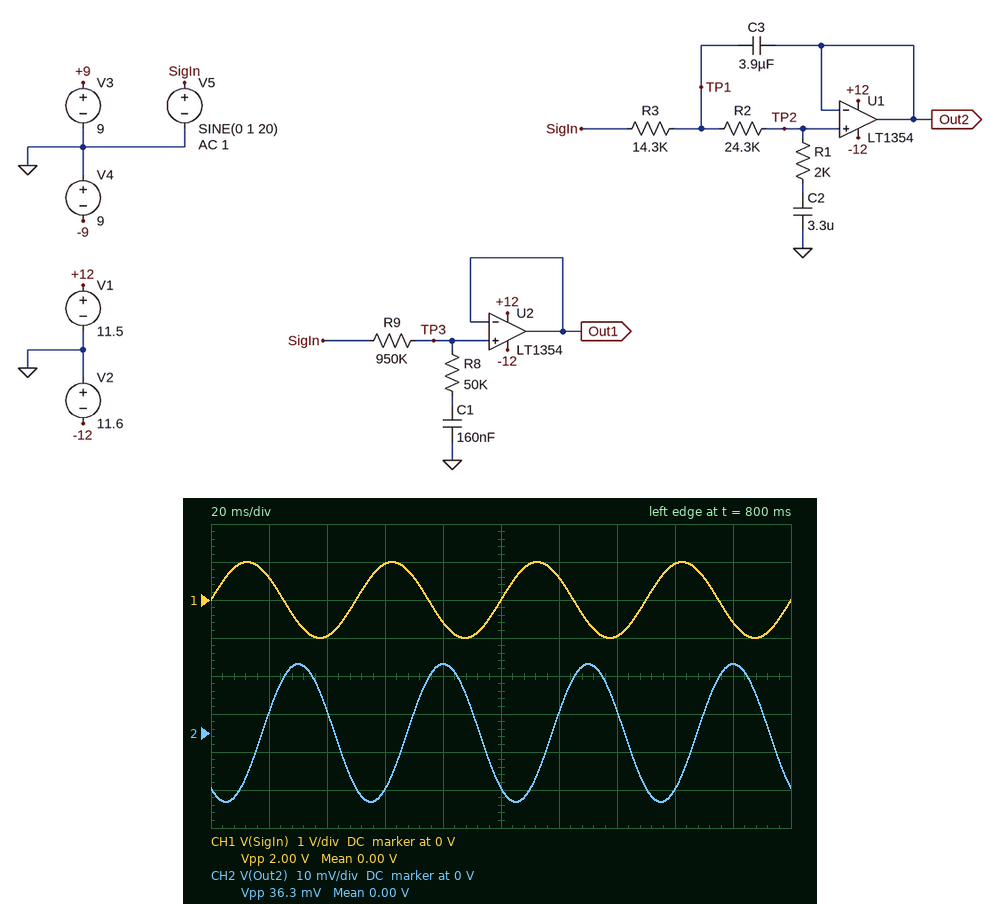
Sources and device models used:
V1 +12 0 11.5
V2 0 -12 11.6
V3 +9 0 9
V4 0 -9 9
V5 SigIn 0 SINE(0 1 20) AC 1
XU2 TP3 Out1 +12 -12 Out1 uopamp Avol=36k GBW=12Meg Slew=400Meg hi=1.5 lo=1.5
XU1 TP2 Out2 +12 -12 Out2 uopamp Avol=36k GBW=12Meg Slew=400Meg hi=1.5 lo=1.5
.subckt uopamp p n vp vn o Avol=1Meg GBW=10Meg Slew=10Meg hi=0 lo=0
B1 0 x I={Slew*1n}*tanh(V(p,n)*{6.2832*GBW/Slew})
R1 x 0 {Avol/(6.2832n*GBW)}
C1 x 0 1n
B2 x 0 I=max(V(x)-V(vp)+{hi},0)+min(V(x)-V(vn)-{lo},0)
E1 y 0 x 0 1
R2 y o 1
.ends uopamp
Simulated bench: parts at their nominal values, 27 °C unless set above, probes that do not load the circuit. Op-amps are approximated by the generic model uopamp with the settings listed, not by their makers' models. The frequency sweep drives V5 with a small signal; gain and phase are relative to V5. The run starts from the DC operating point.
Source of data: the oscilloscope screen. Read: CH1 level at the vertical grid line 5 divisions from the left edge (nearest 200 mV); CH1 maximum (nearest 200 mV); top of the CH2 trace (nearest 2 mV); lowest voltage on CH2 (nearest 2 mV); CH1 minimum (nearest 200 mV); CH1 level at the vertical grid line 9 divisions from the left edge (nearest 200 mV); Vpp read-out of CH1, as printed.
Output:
0 V
1.0 V
18 mV
-18 mV
-1.0 V
-600 mV
2.00 V
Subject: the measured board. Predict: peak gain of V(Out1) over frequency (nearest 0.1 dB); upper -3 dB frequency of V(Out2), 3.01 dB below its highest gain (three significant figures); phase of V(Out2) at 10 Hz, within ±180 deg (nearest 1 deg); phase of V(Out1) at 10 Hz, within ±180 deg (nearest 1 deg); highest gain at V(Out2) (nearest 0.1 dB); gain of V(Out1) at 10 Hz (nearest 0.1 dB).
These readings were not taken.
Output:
0 dB
1.53 Hz
-131 deg
-58 deg
0 dB
-19.1 dB
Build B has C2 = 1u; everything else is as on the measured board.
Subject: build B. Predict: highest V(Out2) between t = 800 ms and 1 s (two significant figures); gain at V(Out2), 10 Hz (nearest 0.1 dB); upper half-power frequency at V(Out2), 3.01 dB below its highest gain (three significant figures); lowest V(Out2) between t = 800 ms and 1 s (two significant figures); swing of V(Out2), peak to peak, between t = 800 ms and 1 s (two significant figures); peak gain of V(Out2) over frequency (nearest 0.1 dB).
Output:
49 mV
-14.0 dB
4.96 Hz
-49 mV
98 mV
0.7 dB
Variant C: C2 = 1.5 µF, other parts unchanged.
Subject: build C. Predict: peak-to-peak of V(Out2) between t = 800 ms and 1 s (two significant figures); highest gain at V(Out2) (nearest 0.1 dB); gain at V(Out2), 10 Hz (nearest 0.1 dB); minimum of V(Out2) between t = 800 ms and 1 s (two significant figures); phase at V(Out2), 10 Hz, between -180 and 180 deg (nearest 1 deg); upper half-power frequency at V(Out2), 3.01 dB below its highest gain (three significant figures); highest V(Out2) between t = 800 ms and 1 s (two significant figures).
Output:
67 mV
0 dB
-17.9 dB
-33 mV
-141 deg
3.68 Hz
33 mV
